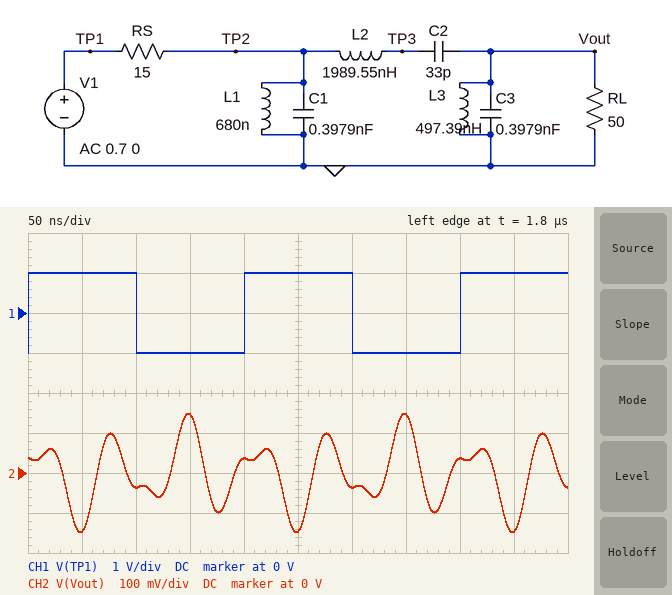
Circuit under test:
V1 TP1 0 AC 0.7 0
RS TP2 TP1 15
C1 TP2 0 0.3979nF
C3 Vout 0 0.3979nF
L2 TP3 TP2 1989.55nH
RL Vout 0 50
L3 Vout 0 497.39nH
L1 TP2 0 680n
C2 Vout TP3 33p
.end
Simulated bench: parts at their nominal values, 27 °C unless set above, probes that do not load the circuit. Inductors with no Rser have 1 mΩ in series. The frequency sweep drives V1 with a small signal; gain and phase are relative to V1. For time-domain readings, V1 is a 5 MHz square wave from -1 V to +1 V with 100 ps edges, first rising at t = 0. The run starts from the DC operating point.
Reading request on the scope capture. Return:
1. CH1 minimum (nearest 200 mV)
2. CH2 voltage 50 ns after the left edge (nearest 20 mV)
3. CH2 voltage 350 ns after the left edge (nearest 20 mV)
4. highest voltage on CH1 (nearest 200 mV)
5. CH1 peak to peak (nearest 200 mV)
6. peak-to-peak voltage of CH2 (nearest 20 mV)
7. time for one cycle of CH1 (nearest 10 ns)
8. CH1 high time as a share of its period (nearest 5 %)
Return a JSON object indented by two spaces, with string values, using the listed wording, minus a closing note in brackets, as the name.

{
  "CH1 minimum": "-1.0 V",
  "CH2 voltage 50 ns after the left edge": "-140 mV",
  "CH2 voltage 350 ns after the left edge": "140 mV",
  "highest voltage on CH1": "1.0 V",
  "CH1 peak to peak": "2.0 V",
  "peak-to-peak voltage of CH2": "300 mV",
  "time for one cycle of CH1": "200 ns",
  "CH1 high time as a share of its period": "50 %"
}
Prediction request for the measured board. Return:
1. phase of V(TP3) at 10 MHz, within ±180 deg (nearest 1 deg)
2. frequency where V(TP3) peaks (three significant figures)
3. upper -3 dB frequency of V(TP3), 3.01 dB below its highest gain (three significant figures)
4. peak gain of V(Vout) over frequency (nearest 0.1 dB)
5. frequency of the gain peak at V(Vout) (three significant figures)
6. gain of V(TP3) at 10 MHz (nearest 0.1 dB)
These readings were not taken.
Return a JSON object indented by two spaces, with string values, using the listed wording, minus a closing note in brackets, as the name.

{
  "phase of V(TP3) at 10 MHz, within ±180 deg": "-6 deg",
  "frequency where V(TP3) peaks": "20.8 MHz",
  "upper -3 dB frequency of V(TP3), 3.01 dB below its highest gain": "21.7 MHz",
  "peak gain of V(Vout) over frequency": "-0.8 dB",
  "frequency of the gain peak at V(Vout)": "20.8 MHz",
  "gain of V(TP3) at 10 MHz": "2.6 dB"
}
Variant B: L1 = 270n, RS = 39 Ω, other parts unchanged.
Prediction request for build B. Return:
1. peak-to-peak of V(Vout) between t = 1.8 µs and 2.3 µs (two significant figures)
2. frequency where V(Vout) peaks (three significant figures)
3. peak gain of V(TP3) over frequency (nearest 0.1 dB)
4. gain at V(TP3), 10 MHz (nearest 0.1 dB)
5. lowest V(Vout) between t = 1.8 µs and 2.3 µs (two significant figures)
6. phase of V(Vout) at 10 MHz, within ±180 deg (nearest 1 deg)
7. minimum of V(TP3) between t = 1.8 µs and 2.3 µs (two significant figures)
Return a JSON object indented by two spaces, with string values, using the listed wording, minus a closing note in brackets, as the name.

{
  "peak-to-peak of V(Vout) between t = 1.8 µs and 2.3 µs": "240 mV",
  "frequency where V(Vout) peaks": "21.3 MHz",
  "peak gain of V(TP3) over frequency": "15.2 dB",
  "gain at V(TP3), 10 MHz": "-1.3 dB",
  "lowest V(Vout) between t = 1.8 µs and 2.3 µs": "-120 mV",
  "phase of V(Vout) at 10 MHz, within ±180 deg": "152 deg",
  "minimum of V(TP3) between t = 1.8 µs and 2.3 µs": "-1.1 V"
}
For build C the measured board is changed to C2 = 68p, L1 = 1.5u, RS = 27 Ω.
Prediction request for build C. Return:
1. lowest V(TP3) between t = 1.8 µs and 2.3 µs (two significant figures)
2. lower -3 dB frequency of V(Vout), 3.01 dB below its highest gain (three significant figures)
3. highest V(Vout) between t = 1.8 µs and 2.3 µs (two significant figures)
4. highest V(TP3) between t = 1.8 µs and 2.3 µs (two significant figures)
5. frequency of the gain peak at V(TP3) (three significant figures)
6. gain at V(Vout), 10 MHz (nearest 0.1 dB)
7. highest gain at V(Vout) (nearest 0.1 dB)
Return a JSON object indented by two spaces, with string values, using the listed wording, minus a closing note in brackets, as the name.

{
  "lowest V(TP3) between t = 1.8 µs and 2.3 µs": "-2.8 V",
  "lower -3 dB frequency of V(Vout), 3.01 dB below its highest gain": "12.2 MHz",
  "highest V(Vout) between t = 1.8 µs and 2.3 µs": "330 mV",
  "highest V(TP3) between t = 1.8 µs and 2.3 µs": "2.8 V",
  "frequency of the gain peak at V(TP3)": "15.5 MHz",
  "gain at V(Vout), 10 MHz": "-8.9 dB",
  "highest gain at V(Vout)": "-3.7 dB"
}
